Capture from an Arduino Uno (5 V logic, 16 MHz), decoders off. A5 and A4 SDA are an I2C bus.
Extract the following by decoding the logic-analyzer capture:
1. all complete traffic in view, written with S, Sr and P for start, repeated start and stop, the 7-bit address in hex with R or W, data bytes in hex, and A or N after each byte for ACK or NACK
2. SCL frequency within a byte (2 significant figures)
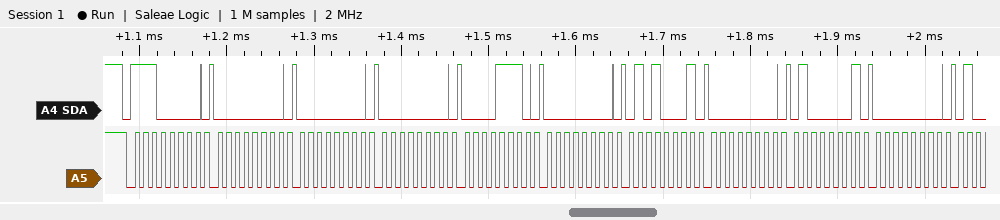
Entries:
S 70W A 00 A 00 A 00 A 0E A 00 A 51 A 00 A 41 A 00 A
100 kHz
